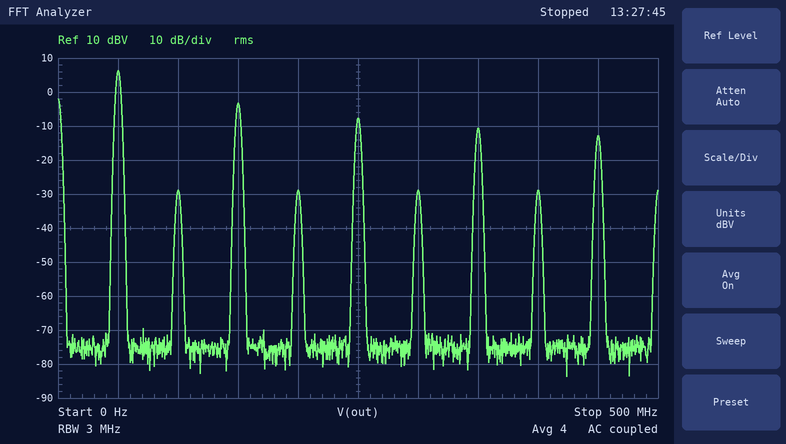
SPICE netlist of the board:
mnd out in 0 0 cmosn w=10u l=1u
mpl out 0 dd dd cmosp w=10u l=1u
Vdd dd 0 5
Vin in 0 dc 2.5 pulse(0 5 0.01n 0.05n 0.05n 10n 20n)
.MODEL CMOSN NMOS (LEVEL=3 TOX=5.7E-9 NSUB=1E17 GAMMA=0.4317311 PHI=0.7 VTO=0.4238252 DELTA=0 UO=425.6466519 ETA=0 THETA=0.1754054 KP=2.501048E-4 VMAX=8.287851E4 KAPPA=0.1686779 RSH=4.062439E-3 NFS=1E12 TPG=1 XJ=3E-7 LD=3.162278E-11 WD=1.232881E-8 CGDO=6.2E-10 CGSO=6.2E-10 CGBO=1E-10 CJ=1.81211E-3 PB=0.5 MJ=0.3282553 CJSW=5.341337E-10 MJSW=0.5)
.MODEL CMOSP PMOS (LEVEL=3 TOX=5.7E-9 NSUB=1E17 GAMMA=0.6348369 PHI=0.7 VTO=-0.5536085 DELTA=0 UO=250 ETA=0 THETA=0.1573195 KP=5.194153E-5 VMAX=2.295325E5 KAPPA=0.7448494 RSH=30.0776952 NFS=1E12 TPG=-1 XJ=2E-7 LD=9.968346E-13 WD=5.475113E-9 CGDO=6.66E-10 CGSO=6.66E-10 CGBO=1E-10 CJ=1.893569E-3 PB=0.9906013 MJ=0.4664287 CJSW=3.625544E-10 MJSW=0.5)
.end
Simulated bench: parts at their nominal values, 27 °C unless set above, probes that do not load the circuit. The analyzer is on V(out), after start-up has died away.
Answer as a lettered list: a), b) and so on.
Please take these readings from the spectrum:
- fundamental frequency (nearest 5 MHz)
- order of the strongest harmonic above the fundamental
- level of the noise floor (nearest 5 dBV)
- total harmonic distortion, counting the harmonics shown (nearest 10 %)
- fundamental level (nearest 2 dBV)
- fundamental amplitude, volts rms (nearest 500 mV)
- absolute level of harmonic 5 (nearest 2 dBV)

a) 50 MHz
b) 3
c) -75 dBV
d) 40 %
e) 6 dBV
f) 2.0 V
g) -8 dBV
